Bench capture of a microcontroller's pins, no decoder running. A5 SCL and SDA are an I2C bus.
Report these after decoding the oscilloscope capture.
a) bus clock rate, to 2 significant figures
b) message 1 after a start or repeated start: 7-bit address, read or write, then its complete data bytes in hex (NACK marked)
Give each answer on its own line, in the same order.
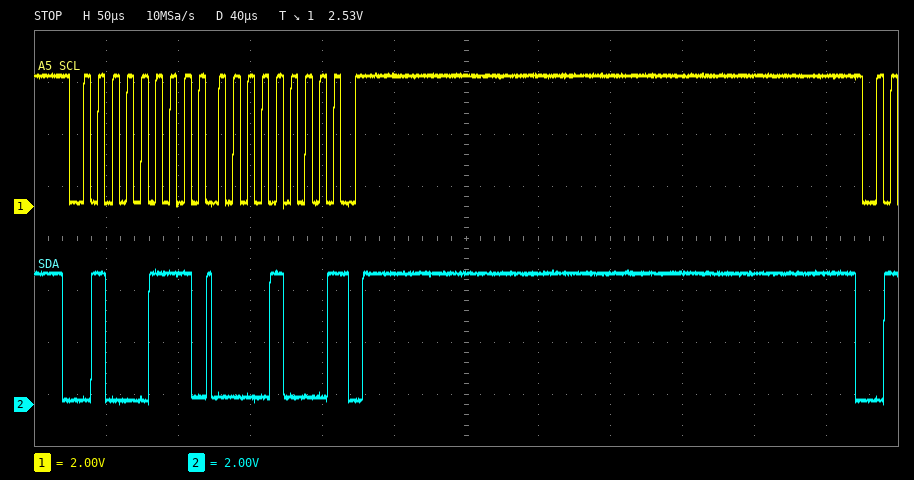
100 kHz
0x23 read: 08 NACK
